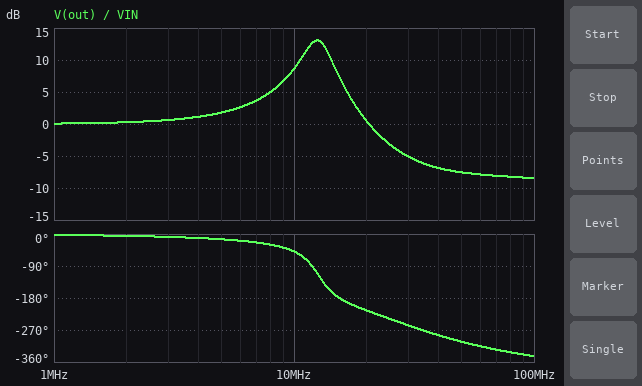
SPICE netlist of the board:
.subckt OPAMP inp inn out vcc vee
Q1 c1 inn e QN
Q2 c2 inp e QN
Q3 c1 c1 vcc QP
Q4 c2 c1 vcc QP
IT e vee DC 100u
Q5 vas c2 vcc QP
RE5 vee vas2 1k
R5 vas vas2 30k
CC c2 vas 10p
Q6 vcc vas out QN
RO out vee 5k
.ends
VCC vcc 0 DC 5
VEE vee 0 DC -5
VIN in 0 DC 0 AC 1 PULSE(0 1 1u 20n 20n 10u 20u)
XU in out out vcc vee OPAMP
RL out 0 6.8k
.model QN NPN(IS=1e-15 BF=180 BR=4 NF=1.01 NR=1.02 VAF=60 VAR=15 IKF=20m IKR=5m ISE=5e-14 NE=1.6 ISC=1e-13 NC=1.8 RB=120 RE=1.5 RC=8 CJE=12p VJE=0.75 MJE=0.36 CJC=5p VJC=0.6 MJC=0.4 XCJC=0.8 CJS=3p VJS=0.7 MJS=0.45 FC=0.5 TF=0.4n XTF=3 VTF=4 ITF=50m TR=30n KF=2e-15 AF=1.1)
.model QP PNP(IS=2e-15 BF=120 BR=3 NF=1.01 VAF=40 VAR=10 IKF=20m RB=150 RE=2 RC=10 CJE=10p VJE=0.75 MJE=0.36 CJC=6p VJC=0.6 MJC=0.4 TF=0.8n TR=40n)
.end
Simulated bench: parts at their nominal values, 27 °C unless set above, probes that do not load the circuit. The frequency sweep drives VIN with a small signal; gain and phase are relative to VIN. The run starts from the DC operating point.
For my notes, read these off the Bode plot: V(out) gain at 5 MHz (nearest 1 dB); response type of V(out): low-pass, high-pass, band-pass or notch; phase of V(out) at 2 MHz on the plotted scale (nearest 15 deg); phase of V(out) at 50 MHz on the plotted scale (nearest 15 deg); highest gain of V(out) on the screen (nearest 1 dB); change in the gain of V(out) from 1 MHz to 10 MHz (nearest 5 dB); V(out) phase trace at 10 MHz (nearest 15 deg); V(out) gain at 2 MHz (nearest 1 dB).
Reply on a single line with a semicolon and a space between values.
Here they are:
2 dB; band-pass; 0 deg; -300 deg; 13 dB; 10 dB; -45 deg; 0 dB
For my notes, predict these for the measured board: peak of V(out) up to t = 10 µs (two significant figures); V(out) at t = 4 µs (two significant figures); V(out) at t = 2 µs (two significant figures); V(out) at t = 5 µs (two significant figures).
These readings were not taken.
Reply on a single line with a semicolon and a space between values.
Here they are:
1.1 V; 1.0 V; 1.0 V; 1.0 V
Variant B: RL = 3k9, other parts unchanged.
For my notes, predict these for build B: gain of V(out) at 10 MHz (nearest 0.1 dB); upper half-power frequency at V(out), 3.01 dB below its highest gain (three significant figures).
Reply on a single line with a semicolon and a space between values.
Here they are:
8.7 dB; 14.2 MHz
